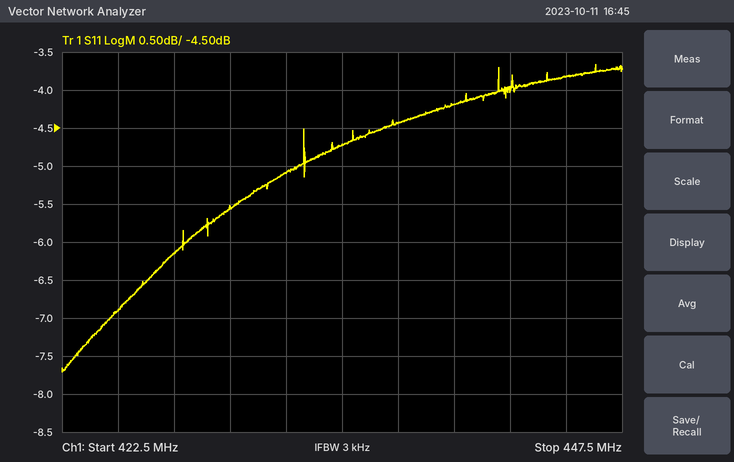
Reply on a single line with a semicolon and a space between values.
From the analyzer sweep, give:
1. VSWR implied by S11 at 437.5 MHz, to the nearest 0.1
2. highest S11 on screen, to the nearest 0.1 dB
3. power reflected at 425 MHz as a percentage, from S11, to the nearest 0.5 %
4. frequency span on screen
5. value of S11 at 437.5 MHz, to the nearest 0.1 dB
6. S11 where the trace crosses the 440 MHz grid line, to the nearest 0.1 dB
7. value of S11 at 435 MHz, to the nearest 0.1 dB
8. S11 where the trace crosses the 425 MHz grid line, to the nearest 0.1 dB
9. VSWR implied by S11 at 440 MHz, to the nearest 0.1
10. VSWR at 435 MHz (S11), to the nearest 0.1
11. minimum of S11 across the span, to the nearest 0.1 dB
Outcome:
4.0; -3.7 dB; 20.5 %; 25 MHz; -4.4 dB; -4.2 dB; -4.7 dB; -6.9 dB; 4.2; 3.8; -7.7 dB
